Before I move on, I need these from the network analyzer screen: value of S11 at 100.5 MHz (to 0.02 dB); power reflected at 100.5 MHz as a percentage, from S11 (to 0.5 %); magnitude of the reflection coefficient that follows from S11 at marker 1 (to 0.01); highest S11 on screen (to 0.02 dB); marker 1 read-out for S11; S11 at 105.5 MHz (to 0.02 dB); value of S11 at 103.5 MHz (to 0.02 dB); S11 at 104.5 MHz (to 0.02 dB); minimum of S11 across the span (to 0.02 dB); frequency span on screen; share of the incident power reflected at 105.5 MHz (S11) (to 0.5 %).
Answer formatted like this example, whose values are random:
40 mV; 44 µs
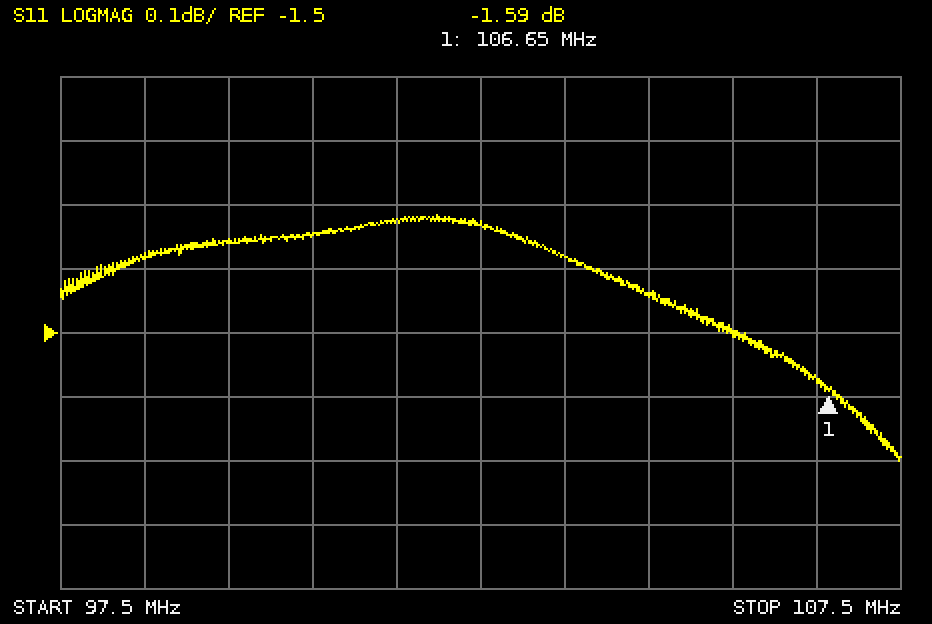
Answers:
-1.34 dB; 73.5 %; 0.83; -1.32 dB; -1.59 dB; -1.50 dB; -1.38 dB; -1.44 dB; -1.70 dB; 10 MHz; 71.0 %
